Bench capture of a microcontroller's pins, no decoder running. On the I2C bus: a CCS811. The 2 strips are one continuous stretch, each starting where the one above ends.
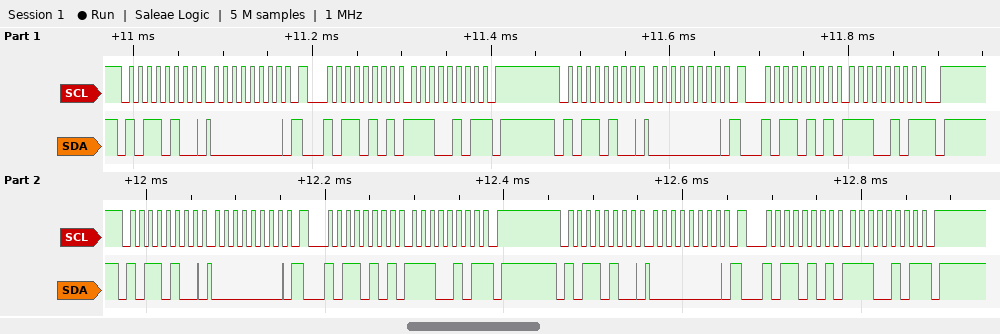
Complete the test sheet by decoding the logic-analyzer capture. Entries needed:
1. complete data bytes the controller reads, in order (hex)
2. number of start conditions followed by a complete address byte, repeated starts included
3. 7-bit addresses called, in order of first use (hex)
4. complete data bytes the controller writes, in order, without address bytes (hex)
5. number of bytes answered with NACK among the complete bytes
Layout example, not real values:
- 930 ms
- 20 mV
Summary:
- E5 E5 E5 E5
- 8
- 0x5A
- 00 00 00 00
- 4
